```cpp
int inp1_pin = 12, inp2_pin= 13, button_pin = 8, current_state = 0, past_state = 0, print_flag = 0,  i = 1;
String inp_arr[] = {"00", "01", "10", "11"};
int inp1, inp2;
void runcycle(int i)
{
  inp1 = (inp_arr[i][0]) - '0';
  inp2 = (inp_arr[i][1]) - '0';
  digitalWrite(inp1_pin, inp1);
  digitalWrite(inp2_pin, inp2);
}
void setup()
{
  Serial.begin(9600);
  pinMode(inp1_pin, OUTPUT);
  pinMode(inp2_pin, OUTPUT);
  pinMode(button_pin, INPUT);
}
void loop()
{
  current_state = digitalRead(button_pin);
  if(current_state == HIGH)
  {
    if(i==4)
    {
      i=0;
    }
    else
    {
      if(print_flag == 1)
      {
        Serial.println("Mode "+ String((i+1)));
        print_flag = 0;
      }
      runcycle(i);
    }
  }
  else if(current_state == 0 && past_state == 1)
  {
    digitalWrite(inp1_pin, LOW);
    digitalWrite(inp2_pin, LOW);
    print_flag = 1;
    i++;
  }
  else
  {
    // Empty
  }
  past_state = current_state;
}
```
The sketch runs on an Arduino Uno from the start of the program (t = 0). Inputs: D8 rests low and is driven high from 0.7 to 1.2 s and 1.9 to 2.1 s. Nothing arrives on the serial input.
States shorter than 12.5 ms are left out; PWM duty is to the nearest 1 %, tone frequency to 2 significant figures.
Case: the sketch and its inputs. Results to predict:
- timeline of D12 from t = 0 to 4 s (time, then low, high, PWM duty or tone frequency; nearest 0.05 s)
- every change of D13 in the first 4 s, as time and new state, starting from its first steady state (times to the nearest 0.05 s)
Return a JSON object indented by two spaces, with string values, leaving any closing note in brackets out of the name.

{
  "timeline of D12 from t = 0 to 4 s": "0 s low; 1.9 s high; 2.1 s low",
  "every change of D13 in the first 4 s, as time and new state, starting from its first steady state": "0 s low; 0.7 s high; 1.2 s low"
}
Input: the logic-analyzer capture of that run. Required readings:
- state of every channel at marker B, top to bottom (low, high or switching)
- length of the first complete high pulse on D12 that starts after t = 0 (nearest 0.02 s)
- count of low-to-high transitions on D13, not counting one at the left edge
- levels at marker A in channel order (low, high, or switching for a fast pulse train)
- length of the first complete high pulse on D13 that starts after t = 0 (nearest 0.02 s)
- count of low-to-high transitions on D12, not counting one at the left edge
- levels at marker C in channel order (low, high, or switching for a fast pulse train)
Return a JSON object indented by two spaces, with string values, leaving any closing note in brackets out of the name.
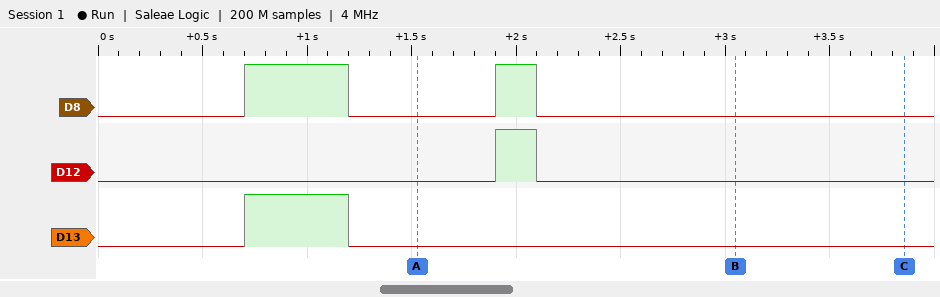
{
  "state of every channel at marker B, top to bottom": "D8 low, D12 low, D13 low",
  "length of the first complete high pulse on D12 that starts after t = 0": "0.20 s",
  "count of low-to-high transitions on D13, not counting one at the left edge": "1",
  "levels at marker A in channel order": "D8 low, D12 low, D13 low",
  "length of the first complete high pulse on D13 that starts after t = 0": "0.50 s",
  "count of low-to-high transitions on D12, not counting one at the left edge": "1",
  "levels at marker C in channel order": "D8 low, D12 low, D13 low"
}
